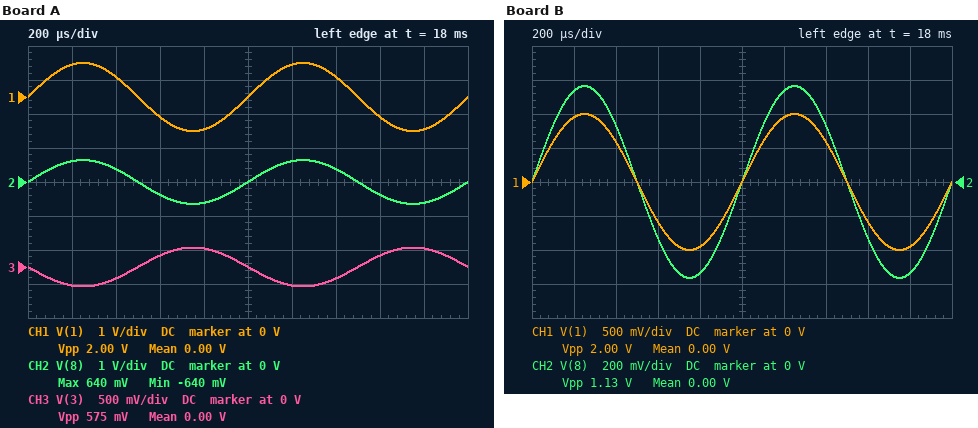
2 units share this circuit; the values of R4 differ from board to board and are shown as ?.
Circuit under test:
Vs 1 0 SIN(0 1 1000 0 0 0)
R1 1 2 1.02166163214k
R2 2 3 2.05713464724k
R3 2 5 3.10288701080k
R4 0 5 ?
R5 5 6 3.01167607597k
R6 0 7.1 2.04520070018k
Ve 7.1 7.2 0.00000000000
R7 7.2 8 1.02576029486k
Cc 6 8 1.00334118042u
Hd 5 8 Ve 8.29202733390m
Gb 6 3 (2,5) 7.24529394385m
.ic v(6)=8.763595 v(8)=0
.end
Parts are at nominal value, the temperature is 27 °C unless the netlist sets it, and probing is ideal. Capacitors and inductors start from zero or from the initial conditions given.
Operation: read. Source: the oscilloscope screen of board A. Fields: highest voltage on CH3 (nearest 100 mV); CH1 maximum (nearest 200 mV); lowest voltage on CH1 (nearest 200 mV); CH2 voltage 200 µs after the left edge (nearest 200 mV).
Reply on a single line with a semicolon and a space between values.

300 mV; 1.0 V; -1.0 V; 600 mV
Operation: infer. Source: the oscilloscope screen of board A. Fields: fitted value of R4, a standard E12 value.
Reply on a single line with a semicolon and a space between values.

3.3 kΩ
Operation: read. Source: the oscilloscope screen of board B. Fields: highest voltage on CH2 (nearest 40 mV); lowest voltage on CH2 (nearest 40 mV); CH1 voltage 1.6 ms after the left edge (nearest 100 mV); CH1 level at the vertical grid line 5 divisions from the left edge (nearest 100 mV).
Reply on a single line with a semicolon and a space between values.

560 mV; -560 mV; -600 mV; 0 V
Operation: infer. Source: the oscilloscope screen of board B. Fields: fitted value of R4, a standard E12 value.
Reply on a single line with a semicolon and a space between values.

1.8 kΩ
